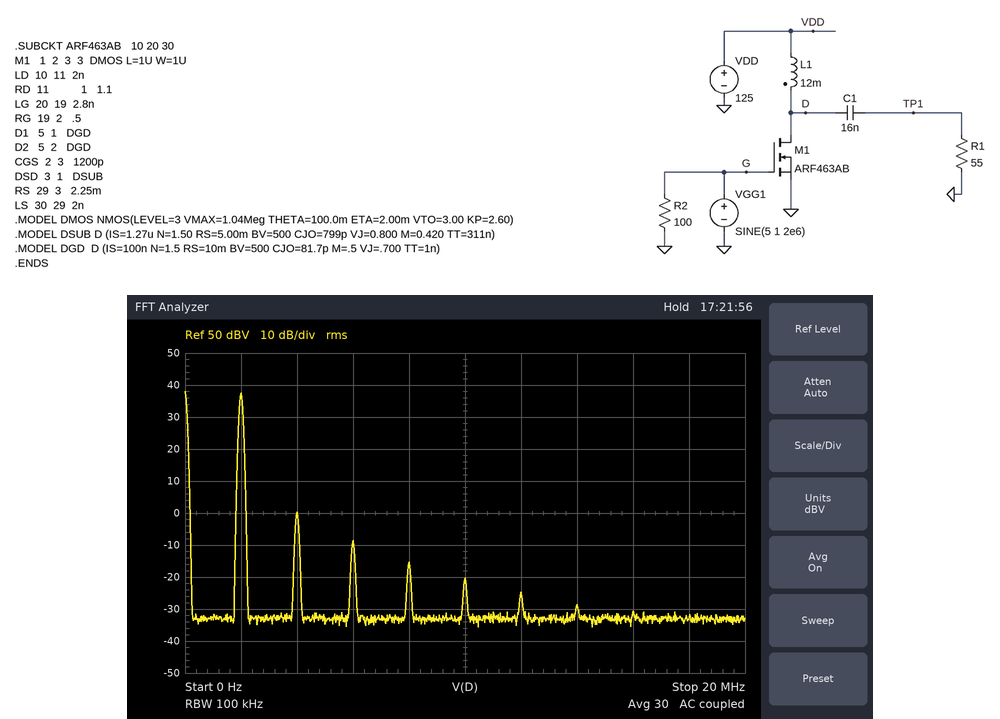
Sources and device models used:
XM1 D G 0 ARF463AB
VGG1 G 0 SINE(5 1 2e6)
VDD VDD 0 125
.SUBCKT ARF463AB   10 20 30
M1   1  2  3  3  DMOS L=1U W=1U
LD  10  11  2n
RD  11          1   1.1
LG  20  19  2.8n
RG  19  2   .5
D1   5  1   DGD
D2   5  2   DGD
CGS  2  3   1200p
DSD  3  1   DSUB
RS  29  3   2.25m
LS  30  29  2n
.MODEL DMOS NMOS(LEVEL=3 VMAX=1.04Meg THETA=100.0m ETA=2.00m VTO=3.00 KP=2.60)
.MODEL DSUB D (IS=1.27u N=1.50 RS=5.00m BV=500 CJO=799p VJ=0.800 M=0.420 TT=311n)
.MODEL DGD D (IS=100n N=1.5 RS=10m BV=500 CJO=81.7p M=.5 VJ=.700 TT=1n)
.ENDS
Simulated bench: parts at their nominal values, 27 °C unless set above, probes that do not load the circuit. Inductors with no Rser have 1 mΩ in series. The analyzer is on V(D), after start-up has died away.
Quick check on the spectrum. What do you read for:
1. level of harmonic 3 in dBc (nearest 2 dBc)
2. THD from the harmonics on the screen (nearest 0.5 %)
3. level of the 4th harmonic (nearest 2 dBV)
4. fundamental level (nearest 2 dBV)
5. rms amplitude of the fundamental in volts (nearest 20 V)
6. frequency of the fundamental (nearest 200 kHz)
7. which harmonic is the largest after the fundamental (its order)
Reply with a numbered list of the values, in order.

1. -46 dBc
2. 1.5 %
3. -16 dBV
4. 38 dBV
5. 80 V
6. 2.0 MHz
7. 2
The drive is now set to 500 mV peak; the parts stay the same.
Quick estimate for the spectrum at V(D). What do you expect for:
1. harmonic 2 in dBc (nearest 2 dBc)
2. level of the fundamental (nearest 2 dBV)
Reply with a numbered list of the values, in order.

1. -44 dBc
2. 32 dBV
